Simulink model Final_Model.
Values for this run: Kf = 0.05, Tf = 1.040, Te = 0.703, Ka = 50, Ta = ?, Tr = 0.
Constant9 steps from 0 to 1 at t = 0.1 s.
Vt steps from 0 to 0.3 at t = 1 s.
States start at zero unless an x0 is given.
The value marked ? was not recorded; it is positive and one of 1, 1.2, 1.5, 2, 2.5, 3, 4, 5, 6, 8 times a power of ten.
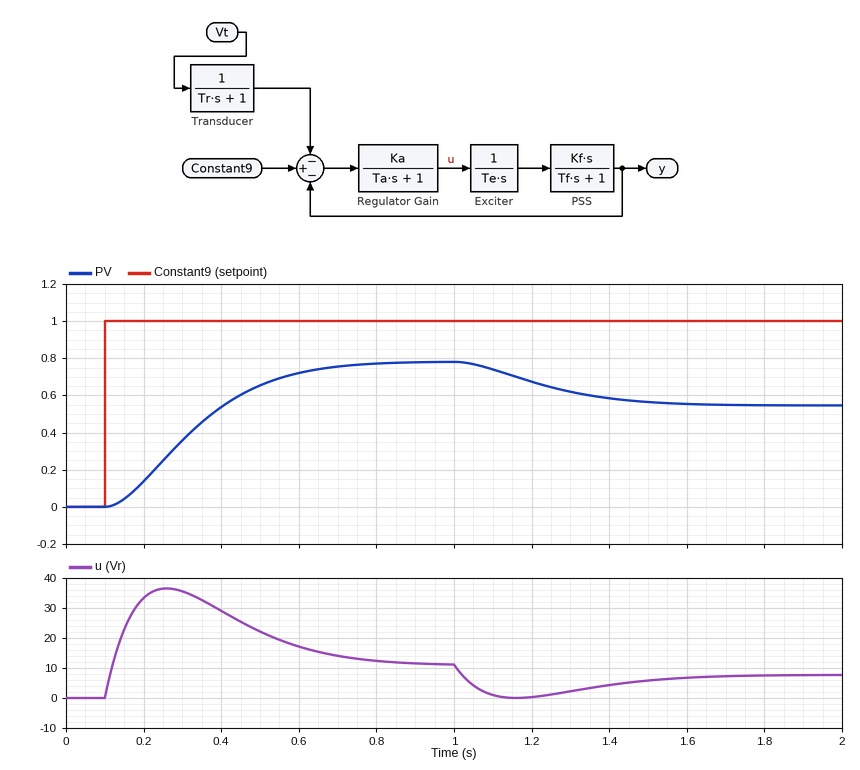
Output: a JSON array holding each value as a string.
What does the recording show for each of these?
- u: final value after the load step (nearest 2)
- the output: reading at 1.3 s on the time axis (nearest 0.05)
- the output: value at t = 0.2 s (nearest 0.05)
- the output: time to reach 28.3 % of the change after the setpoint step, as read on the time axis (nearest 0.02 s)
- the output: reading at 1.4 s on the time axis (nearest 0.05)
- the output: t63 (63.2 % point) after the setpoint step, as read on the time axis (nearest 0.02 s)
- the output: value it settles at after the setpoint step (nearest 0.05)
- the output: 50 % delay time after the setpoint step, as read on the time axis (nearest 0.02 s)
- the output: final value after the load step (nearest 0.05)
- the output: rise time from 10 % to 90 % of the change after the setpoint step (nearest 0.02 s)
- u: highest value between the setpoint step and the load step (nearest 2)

["8", "0.60", "0.15", "0.24 s", "0.60", "0.38 s", "0.80", "0.32 s", "0.55", "0.40 s", "36"]
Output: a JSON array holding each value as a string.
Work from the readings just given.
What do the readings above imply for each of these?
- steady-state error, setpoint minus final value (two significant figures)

["0.20"]
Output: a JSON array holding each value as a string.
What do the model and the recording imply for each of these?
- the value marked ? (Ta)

["0.08"]
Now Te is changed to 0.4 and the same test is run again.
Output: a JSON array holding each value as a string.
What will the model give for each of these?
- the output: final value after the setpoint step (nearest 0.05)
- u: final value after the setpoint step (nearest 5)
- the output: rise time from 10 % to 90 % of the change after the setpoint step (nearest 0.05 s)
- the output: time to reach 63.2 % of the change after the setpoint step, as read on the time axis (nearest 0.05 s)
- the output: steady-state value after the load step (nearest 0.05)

["0.85", "5", "0.25 s", "0.30 s", "0.60"]
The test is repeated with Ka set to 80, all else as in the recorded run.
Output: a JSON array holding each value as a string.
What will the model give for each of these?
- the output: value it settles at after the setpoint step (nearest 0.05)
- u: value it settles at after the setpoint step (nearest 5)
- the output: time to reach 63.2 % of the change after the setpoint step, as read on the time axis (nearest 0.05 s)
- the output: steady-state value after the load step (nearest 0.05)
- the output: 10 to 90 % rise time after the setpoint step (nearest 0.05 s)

["0.85", "10", "0.30 s", "0.60", "0.25 s"]
